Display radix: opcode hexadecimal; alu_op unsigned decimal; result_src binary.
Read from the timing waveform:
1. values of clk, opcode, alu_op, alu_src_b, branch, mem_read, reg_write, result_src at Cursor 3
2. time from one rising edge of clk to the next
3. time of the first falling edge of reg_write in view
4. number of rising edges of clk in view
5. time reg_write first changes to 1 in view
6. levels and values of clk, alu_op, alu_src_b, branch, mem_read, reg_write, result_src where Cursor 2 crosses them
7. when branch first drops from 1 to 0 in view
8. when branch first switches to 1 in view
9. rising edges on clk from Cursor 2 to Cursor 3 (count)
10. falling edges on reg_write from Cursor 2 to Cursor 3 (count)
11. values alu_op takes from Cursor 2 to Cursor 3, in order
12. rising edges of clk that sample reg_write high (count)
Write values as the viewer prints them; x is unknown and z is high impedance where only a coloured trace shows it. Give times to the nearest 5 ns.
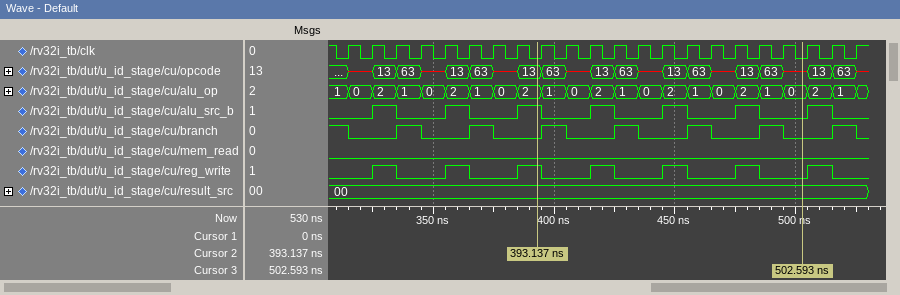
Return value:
clk=0, opcode=x, alu_op=0, alu_src_b=0, branch=0, mem_read=0, reg_write=0, result_src=00
10 ns
335 ns
22
325 ns
clk=0, alu_op=2, alu_src_b=1, branch=0, mem_read=0, reg_write=1, result_src=00
315 ns
335 ns
11
4
2, 1, 0, 2, 1, 0, 2, 1, 0, 2, 1, 0
7
